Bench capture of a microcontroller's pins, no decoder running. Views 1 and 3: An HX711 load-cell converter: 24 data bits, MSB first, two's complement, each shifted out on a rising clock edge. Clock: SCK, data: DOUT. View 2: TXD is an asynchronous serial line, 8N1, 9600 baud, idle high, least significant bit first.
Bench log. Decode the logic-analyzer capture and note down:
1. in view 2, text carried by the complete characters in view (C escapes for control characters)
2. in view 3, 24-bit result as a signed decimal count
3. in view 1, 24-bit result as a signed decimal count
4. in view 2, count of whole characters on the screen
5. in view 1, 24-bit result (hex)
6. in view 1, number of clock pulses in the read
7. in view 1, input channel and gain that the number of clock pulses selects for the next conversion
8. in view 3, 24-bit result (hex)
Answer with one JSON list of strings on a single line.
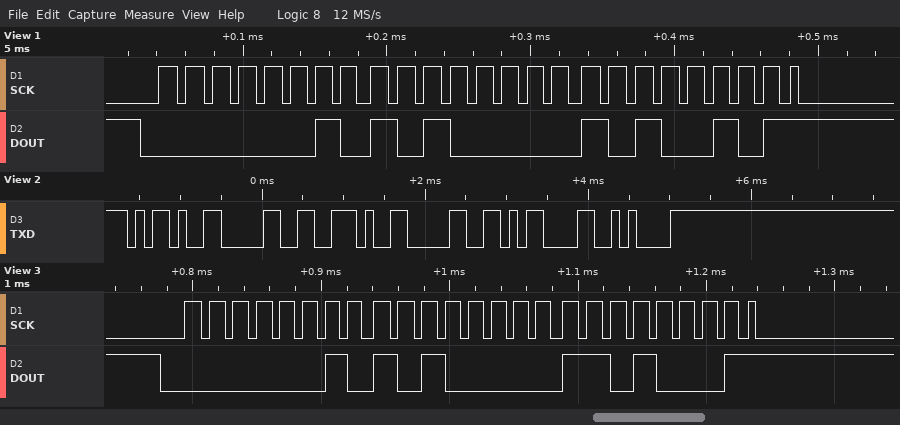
["\"-0.0\\r\\n\"", "172241", "172197", "6", "0x02A0A5", "25", "channel A, gain 128", "0x02A0D1"]
